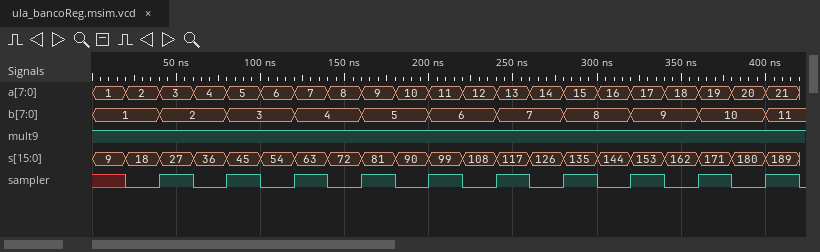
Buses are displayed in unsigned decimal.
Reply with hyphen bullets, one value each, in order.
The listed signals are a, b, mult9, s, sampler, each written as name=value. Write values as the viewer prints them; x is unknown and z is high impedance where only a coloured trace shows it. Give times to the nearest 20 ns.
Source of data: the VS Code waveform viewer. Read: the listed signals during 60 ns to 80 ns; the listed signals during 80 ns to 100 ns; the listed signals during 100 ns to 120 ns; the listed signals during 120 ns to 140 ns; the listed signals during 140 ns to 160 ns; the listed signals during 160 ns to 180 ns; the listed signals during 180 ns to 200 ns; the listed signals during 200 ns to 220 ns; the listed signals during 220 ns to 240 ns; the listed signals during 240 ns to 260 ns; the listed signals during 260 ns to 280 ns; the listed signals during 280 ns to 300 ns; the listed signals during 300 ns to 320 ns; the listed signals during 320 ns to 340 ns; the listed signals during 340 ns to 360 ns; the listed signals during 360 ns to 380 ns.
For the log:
- a=4, b=2, mult9=1, s=36, sampler=0
- a=5, b=3, mult9=1, s=45, sampler=1
- a=6, b=3, mult9=1, s=54, sampler=0
- a=7, b=4, mult9=1, s=63, sampler=1
- a=8, b=4, mult9=1, s=72, sampler=0
- a=9, b=5, mult9=1, s=81, sampler=1
- a=10, b=5, mult9=1, s=90, sampler=0
- a=11, b=6, mult9=1, s=99, sampler=1
- a=12, b=6, mult9=1, s=108, sampler=0
- a=13, b=7, mult9=1, s=117, sampler=1
- a=14, b=7, mult9=1, s=126, sampler=0
- a=15, b=8, mult9=1, s=135, sampler=1
- a=16, b=8, mult9=1, s=144, sampler=0
- a=17, b=9, mult9=1, s=153, sampler=1
- a=18, b=9, mult9=1, s=162, sampler=0
- a=19, b=10, mult9=1, s=171, sampler=1
